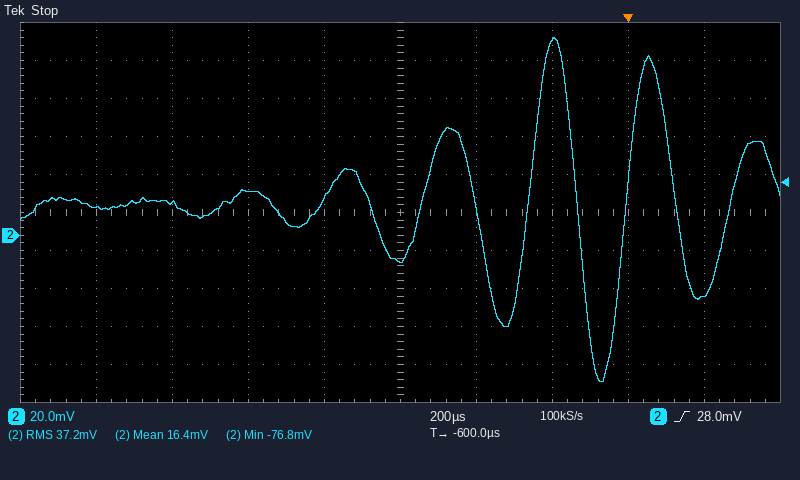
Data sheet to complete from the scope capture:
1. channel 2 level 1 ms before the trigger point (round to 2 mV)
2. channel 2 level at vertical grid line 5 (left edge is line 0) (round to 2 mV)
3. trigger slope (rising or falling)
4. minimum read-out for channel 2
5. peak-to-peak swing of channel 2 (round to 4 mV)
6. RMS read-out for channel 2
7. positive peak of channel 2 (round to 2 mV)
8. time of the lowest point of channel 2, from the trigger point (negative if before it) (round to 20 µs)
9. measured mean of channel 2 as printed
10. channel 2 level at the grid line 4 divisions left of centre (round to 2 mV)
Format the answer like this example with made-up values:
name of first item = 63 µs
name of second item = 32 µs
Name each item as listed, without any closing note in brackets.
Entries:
channel 2 level 1 ms before the trigger point = 24 mV
channel 2 level at vertical grid line 5 (left edge is line 0) = -14 mV
trigger slope = rising
minimum read-out for channel 2 = -76.8 mV
peak-to-peak swing of channel 2 = 180 mV
RMS read-out for channel 2 = 37.2 mV
positive peak of channel 2 = 104 mV
time of the lowest point of channel 2, from the trigger point (negative if before it) = -80 µs
measured mean of channel 2 as printed = 16.4 mV
channel 2 level at the grid line 4 divisions left of centre = 14 mV
